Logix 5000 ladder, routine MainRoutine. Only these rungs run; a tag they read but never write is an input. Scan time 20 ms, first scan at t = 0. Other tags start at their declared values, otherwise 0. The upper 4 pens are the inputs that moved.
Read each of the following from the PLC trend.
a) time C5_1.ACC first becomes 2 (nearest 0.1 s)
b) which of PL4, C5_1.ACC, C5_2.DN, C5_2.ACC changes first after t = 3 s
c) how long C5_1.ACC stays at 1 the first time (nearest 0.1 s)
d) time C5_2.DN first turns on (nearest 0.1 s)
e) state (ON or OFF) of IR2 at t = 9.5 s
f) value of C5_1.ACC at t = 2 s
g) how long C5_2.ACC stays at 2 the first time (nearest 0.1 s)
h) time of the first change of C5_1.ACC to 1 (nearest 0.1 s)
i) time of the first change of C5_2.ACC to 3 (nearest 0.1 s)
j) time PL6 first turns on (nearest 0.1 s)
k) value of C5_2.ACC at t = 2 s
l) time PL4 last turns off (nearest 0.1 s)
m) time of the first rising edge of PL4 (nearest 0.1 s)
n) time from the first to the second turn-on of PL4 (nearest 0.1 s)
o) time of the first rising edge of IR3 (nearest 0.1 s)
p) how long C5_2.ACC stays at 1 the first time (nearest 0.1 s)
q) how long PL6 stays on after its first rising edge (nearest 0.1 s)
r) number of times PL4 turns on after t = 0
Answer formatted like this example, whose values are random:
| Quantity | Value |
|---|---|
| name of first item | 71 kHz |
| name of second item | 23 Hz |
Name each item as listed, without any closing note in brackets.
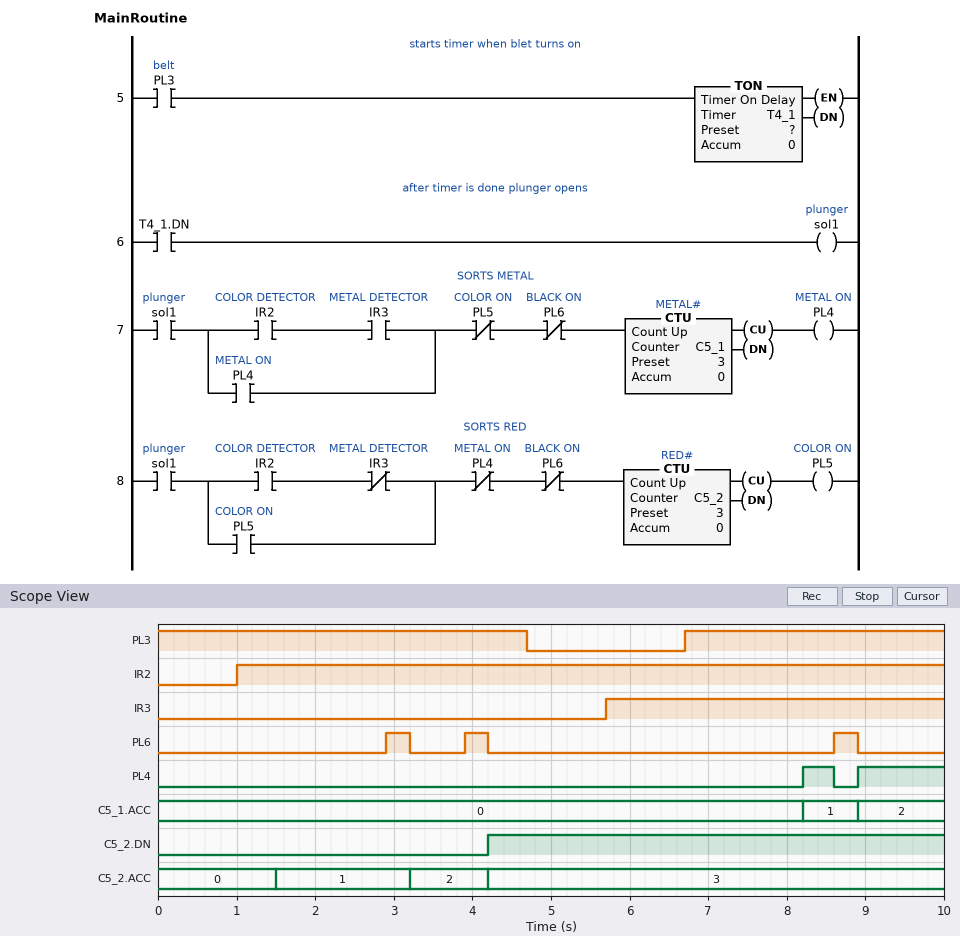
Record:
| Quantity | Value |
|---|---|
| time C5_1.ACC first becomes 2 | 8.9 s |
| which of PL4, C5_1.ACC, C5_2.DN, C5_2.ACC changes first after t = 3 s | C5_2.ACC |
| how long C5_1.ACC stays at 1 the first time | 0.7 s |
| time C5_2.DN first turns on | 4.2 s |
| state (ON or OFF) of IR2 at t = 9.5 s | ON |
| value of C5_1.ACC at t = 2 s | 0 |
| how long C5_2.ACC stays at 2 the first time | 1.0 s |
| time of the first change of C5_1.ACC to 1 | 8.2 s |
| time of the first change of C5_2.ACC to 3 | 4.2 s |
| time PL6 first turns on | 2.9 s |
| value of C5_2.ACC at t = 2 s | 1 |
| time PL4 last turns off | 8.6 s |
| time of the first rising edge of PL4 | 8.2 s |
| time from the first to the second turn-on of PL4 | 0.7 s |
| time of the first rising edge of IR3 | 5.7 s |
| how long C5_2.ACC stays at 1 the first time | 1.7 s |
| how long PL6 stays on after its first rising edge | 0.3 s |
| number of times PL4 turns on after t = 0 | 2 |
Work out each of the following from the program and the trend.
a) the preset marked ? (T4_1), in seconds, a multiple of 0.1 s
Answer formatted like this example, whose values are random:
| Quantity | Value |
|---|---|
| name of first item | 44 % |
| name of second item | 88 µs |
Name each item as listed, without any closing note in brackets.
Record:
| Quantity | Value |
|---|---|
| the preset marked ? (T4_1), in seconds, a multiple of 0.1 s | 1.5 s |
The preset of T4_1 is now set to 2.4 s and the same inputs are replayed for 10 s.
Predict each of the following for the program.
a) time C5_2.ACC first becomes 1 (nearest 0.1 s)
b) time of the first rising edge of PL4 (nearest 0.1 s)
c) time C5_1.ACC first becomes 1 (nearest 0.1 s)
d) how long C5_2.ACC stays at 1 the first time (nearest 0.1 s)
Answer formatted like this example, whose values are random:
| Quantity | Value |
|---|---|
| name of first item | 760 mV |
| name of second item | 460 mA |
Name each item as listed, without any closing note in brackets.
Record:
| Quantity | Value |
|---|---|
| time C5_2.ACC first becomes 1 | 2.4 s |
| time of the first rising edge of PL4 | 9.1 s |
| time C5_1.ACC first becomes 1 | 9.1 s |
| how long C5_2.ACC stays at 1 the first time | 0.8 s |
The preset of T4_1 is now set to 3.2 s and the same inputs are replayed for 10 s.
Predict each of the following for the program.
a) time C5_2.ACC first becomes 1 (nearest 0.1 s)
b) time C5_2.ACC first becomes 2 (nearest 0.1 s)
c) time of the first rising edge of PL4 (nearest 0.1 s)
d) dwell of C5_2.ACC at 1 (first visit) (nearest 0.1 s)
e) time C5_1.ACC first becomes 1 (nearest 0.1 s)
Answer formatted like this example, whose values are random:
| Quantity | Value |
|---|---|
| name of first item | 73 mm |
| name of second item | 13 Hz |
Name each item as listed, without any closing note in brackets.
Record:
| Quantity | Value |
|---|---|
| time C5_2.ACC first becomes 1 | 3.2 s |
| time C5_2.ACC first becomes 2 | 4.2 s |
| time of the first rising edge of PL4 | 9.9 s |
| dwell of C5_2.ACC at 1 (first visit) | 1.0 s |
| time C5_1.ACC first becomes 1 | 9.9 s |
